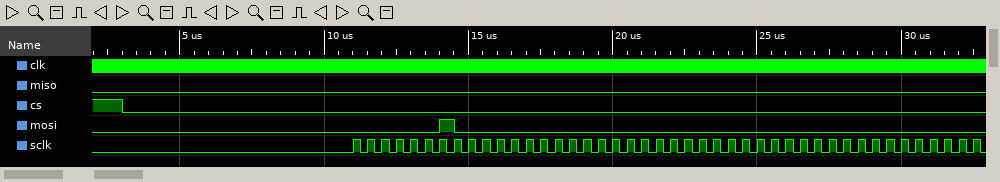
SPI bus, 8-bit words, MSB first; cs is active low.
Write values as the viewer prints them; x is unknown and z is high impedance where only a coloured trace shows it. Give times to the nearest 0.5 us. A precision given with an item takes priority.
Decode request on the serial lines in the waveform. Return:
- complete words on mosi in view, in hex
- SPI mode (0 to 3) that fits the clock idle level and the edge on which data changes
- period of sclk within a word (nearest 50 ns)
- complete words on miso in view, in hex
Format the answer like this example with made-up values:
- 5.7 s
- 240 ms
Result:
- 02, 00, 00, 00, 00
- 1
- 500 ns
- 00, 00, 00, 00, 00
